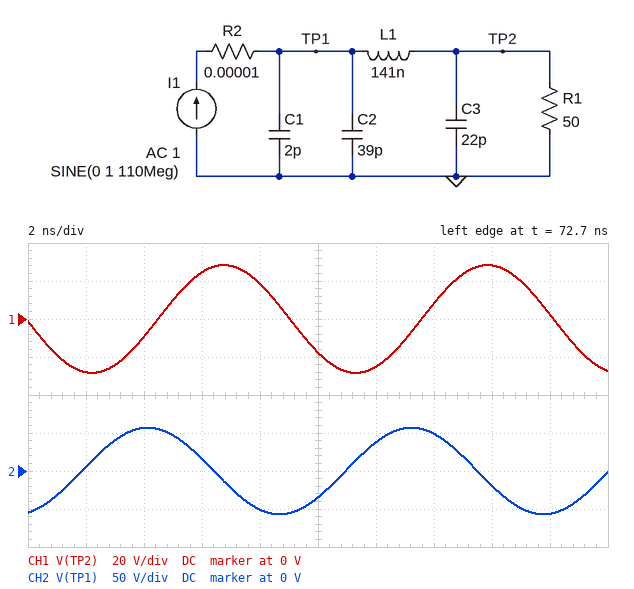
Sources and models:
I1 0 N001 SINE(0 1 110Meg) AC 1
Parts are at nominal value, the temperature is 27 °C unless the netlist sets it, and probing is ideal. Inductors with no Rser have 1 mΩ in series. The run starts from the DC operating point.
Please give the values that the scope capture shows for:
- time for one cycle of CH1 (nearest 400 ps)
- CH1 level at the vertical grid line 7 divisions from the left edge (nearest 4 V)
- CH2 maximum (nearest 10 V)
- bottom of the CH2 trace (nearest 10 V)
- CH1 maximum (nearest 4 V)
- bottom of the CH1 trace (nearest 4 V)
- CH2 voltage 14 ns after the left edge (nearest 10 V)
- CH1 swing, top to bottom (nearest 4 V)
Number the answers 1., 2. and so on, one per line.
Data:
1. 9.2 ns
2. 8 V
3. 60 V
4. -60 V
5. 28 V
6. -28 V
7. 50 V
8. 56 V
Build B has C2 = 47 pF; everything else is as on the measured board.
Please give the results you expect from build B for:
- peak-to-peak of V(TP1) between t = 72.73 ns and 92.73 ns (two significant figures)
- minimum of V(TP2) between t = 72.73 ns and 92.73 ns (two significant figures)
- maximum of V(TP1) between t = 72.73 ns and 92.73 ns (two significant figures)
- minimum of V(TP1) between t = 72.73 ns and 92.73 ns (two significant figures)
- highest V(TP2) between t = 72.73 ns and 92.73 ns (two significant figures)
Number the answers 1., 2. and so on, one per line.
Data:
1. 87 V
2. -22 V
3. 44 V
4. -44 V
5. 22 V
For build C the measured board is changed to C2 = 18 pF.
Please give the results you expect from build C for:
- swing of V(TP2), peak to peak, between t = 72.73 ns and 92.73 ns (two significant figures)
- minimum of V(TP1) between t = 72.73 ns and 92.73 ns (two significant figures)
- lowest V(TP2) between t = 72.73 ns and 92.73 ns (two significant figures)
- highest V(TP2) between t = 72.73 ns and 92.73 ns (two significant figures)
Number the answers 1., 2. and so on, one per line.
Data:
1. 180 V
2. -180 V
3. -91 V
4. 91 V
